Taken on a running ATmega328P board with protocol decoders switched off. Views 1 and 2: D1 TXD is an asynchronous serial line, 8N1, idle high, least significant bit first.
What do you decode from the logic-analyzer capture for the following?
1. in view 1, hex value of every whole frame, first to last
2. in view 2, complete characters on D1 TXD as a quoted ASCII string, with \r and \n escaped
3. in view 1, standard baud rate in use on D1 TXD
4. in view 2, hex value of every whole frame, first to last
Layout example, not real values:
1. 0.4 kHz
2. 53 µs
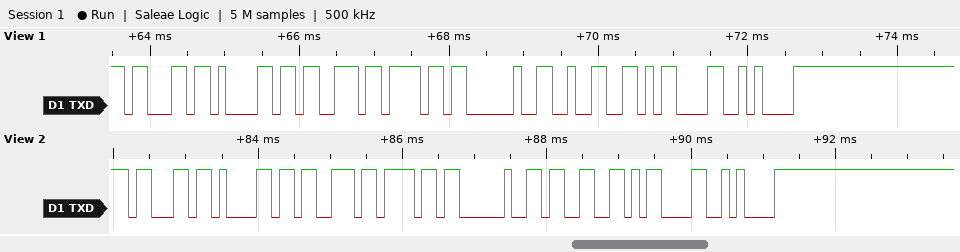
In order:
1. 0x63 0x61 0x73 0x6F 0x20 0x32 0x0D 0x0A
2. "caso 3\r\n"
3. 9600 baud
4. 63 61 73 6F 20 33 0D 0A
